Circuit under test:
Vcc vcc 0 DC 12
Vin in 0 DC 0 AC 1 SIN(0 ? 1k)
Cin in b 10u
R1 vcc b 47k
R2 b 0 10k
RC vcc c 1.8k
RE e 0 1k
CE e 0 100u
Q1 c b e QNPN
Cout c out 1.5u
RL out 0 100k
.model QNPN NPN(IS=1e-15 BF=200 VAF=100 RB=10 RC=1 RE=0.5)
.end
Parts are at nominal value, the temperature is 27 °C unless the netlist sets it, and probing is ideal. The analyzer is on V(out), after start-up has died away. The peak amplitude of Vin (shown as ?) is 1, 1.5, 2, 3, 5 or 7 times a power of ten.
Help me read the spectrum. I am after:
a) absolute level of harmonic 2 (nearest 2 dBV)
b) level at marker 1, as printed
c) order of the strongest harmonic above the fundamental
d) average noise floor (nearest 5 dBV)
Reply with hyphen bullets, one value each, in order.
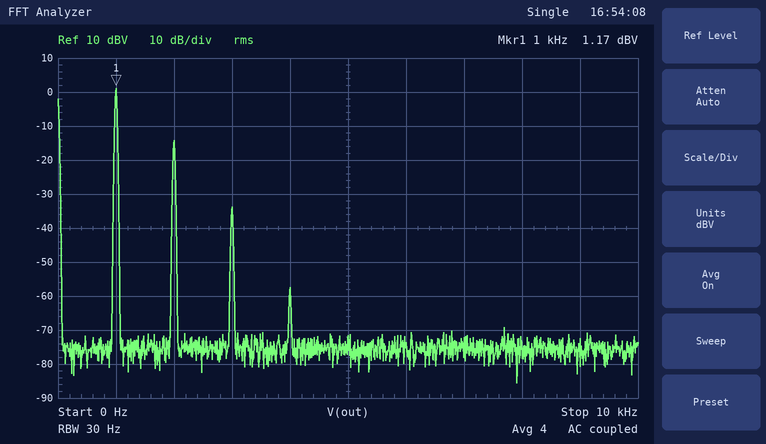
- -14 dBV
- 1.17 dBV
- 2
- -75 dBV
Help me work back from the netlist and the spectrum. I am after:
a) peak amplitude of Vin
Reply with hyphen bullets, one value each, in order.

- 20 mV
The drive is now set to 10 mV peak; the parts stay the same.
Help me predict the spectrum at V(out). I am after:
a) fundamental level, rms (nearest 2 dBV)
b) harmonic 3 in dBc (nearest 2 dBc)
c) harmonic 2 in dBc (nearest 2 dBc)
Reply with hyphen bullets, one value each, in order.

- -4 dBV
- -46 dBc
- -22 dBc
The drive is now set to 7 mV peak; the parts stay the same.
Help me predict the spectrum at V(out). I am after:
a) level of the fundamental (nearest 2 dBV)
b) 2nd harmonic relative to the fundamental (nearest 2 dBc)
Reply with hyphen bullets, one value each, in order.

- -8 dBV
- -24 dBc
